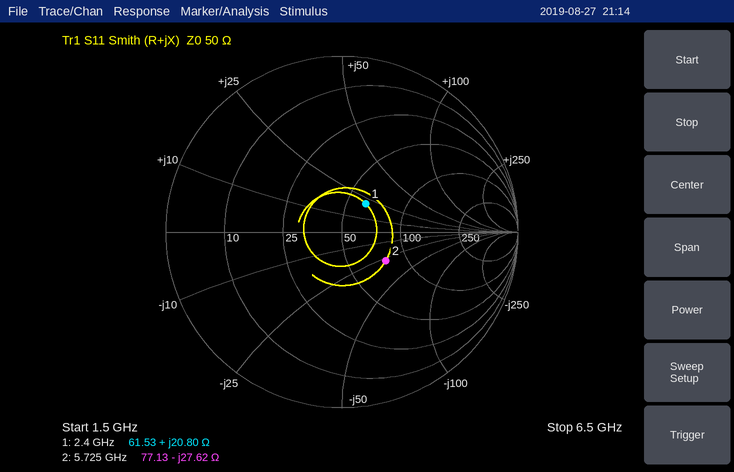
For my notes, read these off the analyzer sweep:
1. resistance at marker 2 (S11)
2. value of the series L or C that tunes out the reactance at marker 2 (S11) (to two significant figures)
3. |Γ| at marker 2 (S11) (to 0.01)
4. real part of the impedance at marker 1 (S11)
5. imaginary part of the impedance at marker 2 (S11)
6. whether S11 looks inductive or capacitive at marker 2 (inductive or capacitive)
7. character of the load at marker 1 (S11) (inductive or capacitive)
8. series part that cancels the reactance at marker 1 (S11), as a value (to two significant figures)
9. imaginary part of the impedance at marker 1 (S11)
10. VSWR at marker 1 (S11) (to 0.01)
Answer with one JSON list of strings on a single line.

["77.13 Ω", "770 pH", "0.30", "61.53 Ω", "-27.62 Ω", "capacitive", "inductive", "3.2 pF", "+20.80 Ω", "1.53"]
